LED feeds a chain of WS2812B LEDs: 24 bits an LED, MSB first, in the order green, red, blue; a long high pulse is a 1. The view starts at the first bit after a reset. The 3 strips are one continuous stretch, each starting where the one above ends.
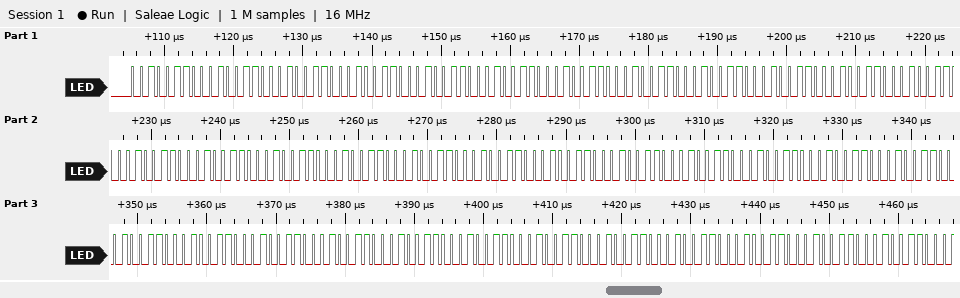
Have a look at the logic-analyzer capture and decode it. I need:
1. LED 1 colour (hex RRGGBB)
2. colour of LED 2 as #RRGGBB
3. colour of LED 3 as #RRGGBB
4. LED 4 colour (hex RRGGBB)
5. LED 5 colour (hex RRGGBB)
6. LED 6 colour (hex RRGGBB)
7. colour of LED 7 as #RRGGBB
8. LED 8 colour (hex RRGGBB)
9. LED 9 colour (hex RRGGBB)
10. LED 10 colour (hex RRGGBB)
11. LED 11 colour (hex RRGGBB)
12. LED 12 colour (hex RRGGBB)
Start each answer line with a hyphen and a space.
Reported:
- #262626
- #262626
- #262626
- #262626
- #262626
- #262626
- #262626
- #262626
- #262626
- #262626
- #262626
- #262626
